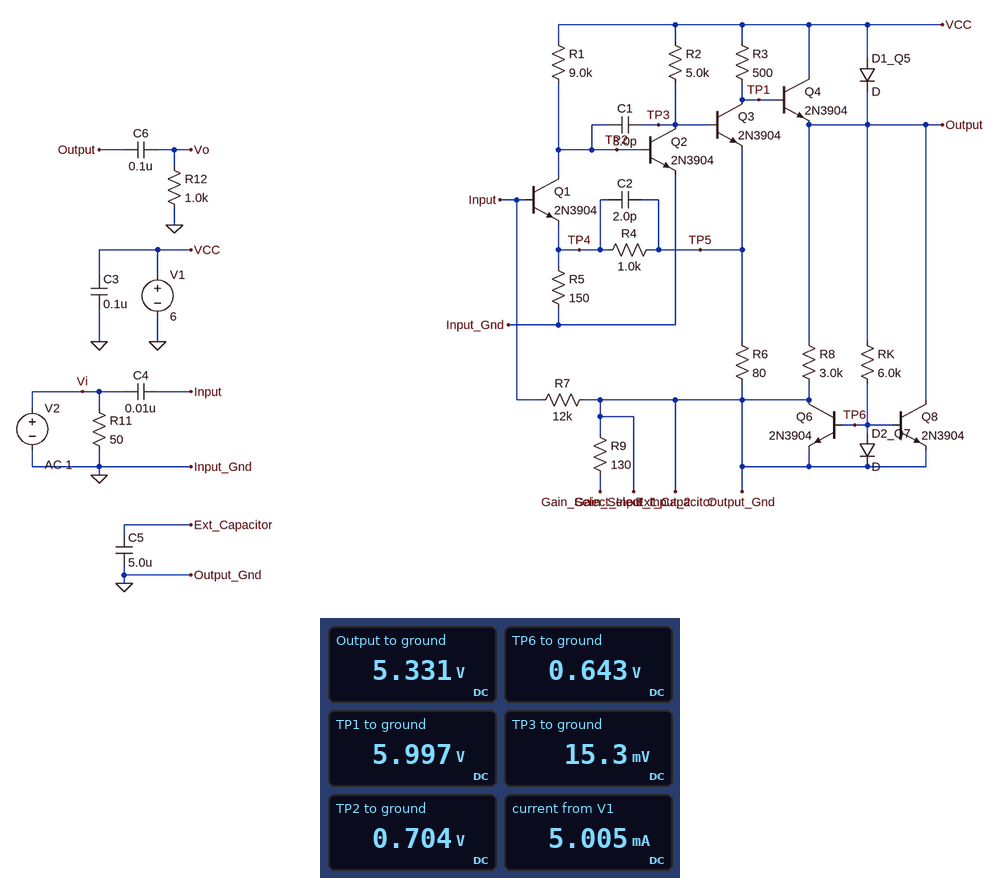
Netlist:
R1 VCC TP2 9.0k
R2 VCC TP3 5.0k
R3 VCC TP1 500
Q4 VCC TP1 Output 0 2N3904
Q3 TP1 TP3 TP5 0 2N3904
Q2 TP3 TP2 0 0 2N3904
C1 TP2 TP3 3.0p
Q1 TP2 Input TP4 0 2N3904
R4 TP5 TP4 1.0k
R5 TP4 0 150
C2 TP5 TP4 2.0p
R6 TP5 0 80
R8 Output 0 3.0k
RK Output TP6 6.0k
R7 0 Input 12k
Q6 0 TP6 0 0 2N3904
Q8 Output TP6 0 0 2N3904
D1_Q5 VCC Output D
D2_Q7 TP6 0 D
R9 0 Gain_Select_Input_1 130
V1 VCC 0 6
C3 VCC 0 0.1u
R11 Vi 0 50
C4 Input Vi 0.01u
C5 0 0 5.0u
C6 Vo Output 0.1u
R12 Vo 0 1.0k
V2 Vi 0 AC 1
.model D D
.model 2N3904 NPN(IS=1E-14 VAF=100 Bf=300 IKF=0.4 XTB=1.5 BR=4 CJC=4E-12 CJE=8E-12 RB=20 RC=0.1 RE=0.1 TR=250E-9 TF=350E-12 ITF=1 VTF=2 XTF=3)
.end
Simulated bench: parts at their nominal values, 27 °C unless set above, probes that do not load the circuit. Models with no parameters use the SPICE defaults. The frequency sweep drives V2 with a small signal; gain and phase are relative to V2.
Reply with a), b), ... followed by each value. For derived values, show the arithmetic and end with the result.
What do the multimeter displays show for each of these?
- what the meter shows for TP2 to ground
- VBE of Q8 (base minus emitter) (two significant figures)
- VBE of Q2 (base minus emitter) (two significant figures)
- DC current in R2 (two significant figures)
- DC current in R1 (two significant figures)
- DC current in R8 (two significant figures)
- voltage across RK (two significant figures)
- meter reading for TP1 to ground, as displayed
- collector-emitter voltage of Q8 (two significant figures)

a) 0.704 V
b) 643 mV = 640 mV
c) 704 mV = 700 mV
d) (6 V - 15.3 mV) / 5 kΩ = 1.2 mA
e) (6 V - 704 mV) / 9 kΩ = 590 µA
f) (5.331 V) / 3 kΩ = 1.8 mA
g) 5.331 V - 643 mV = 4.7 V
h) 5.997 V
i) 5.331 V = 5.3 V
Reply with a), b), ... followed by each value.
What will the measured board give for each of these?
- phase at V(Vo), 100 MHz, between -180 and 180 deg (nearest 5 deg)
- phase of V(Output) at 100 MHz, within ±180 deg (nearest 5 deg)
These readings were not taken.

a) 110 deg
b) 110 deg
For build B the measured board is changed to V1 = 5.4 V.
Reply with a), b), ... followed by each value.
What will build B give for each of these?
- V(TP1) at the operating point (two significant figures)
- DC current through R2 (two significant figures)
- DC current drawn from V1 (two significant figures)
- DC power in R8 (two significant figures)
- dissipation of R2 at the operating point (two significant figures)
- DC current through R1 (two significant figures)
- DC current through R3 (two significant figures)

a) 5.4 V
b) 1.1 mA
c) 4.4 mA
d) 7.5 mW
e) 5.8 mW
f) 520 µA
g) 4.5 µA
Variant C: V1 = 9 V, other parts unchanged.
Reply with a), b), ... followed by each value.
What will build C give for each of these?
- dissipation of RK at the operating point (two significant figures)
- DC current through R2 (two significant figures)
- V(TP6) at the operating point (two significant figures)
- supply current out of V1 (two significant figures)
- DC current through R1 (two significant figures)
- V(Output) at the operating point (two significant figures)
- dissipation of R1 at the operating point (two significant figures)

a) 9.8 mW
b) 1.8 mA
c) 660 mV
d) 7.9 mA
e) 920 µA
f) 8.3 V
g) 7.6 mW
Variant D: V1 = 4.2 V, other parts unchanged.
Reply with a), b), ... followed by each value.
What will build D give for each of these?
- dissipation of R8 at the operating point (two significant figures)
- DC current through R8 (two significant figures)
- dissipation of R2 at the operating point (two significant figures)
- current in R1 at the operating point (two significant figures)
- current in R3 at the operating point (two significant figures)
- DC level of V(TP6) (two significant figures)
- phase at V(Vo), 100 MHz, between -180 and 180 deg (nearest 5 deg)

a) 4.2 mW
b) 1.2 mA
c) 3.5 mW
d) 390 µA
e) 3.3 µA
f) 630 mV
g) 105 deg
